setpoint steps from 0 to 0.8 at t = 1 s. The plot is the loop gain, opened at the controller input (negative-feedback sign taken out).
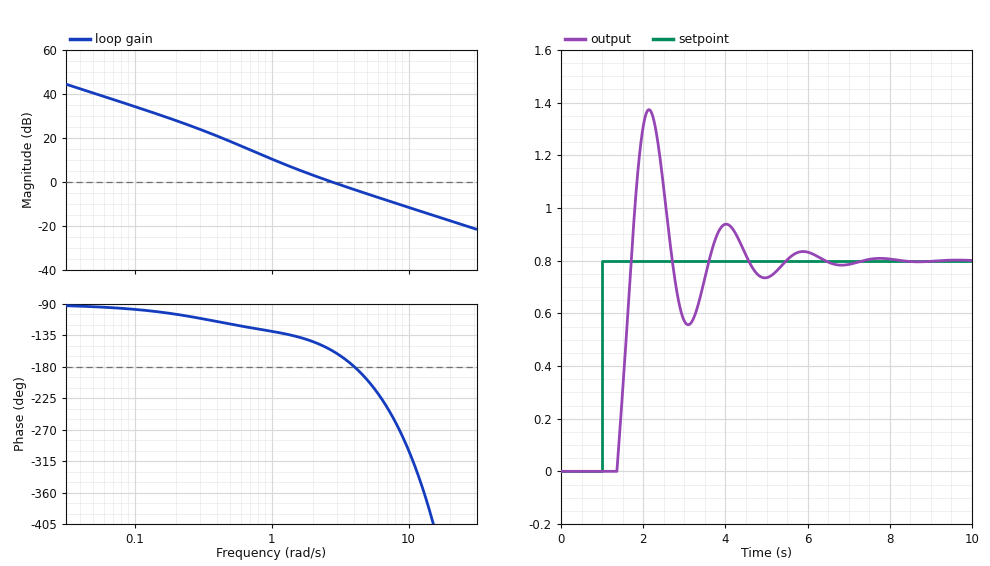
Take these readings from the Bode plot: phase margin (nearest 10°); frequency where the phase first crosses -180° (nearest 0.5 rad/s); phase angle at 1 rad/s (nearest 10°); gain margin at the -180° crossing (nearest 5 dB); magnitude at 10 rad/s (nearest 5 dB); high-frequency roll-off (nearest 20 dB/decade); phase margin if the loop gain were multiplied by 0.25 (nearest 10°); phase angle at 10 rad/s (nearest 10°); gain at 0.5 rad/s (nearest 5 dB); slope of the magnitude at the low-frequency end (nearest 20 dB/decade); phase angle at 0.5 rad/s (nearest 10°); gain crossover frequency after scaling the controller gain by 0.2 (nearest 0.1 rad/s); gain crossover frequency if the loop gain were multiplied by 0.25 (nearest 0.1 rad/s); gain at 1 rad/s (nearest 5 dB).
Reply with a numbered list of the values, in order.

1. 20°
2. 4.0 rad/s
3. -130°
4. 5 dB
5. -10 dB
6. -20 dB/decade
7. 50°
8. -300°
9. 20 dB
10. -20 dB/decade
11. -120°
12. 0.7 rad/s
13. 0.9 rad/s
14. 10 dB
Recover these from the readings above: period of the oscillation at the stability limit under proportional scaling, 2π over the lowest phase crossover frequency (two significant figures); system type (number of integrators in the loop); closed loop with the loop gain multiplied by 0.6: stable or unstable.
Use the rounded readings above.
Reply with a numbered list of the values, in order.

1. 1.6 s
2. 1
3. stable
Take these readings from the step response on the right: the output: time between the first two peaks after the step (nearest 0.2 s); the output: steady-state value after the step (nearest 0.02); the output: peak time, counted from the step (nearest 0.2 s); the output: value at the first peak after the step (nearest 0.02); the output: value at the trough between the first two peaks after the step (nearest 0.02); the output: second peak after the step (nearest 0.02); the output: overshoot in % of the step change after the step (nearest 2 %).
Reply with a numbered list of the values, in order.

1. 1.8 s
2. 0.80
3. 1.2 s
4. 1.38
5. 0.56
6. 0.94
7. 72 %
